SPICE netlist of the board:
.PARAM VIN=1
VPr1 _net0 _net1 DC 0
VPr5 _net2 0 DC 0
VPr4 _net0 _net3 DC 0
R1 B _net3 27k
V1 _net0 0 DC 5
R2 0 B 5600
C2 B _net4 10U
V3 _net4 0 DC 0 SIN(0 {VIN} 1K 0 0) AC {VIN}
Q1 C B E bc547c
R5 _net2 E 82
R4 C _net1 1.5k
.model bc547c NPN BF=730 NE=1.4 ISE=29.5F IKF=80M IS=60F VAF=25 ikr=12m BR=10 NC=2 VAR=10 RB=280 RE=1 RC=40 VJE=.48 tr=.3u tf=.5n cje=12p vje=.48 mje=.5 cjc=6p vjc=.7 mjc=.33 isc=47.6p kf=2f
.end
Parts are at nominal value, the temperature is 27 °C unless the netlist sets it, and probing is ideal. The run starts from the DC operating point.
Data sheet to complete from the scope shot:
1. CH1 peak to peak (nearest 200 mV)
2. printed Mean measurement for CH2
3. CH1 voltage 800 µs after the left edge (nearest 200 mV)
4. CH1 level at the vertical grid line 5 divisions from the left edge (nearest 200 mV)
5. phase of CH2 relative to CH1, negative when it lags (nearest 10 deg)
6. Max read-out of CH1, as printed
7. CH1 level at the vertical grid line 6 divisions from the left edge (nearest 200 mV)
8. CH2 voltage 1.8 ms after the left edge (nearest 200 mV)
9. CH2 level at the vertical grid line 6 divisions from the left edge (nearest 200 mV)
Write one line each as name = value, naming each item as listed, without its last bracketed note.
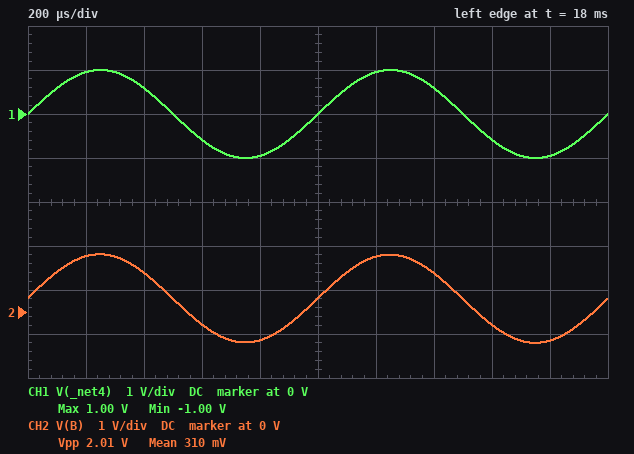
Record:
CH1 peak to peak = 2.0 V
printed Mean measurement for CH2 = 310 mV
CH1 voltage 800 µs after the left edge = -1.0 V
CH1 level at the vertical grid line 5 divisions from the left edge = 0 V
phase of CH2 relative to CH1, negative when it lags = 0 deg
Max read-out of CH1, as printed = 1.00 V
CH1 level at the vertical grid line 6 divisions from the left edge = 1.0 V
CH2 voltage 1.8 ms after the left edge = -600 mV
CH2 level at the vertical grid line 6 divisions from the left edge = 1.2 V
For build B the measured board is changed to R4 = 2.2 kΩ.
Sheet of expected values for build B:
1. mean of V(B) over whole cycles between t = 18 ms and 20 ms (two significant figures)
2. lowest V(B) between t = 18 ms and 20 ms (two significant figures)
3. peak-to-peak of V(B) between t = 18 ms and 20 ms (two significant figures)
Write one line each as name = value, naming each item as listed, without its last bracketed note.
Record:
mean of V(B) over whole cycles between t = 18 ms and 20 ms = 250 mV
lowest V(B) between t = 18 ms and 20 ms = -760 mV
peak-to-peak of V(B) between t = 18 ms and 20 ms = 2.0 V
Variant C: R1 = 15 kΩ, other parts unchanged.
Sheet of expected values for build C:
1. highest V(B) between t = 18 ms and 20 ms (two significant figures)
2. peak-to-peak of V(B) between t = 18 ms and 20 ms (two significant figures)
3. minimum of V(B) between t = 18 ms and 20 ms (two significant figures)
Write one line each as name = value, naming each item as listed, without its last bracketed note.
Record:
highest V(B) between t = 18 ms and 20 ms = 1.4 V
peak-to-peak of V(B) between t = 18 ms and 20 ms = 2.0 V
minimum of V(B) between t = 18 ms and 20 ms = -580 mV
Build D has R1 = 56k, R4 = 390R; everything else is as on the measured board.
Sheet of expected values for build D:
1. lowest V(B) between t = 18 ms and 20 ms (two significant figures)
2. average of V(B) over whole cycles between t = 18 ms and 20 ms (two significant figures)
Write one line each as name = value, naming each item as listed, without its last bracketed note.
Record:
lowest V(B) between t = 18 ms and 20 ms = -560 mV
average of V(B) over whole cycles between t = 18 ms and 20 ms = 440 mV
